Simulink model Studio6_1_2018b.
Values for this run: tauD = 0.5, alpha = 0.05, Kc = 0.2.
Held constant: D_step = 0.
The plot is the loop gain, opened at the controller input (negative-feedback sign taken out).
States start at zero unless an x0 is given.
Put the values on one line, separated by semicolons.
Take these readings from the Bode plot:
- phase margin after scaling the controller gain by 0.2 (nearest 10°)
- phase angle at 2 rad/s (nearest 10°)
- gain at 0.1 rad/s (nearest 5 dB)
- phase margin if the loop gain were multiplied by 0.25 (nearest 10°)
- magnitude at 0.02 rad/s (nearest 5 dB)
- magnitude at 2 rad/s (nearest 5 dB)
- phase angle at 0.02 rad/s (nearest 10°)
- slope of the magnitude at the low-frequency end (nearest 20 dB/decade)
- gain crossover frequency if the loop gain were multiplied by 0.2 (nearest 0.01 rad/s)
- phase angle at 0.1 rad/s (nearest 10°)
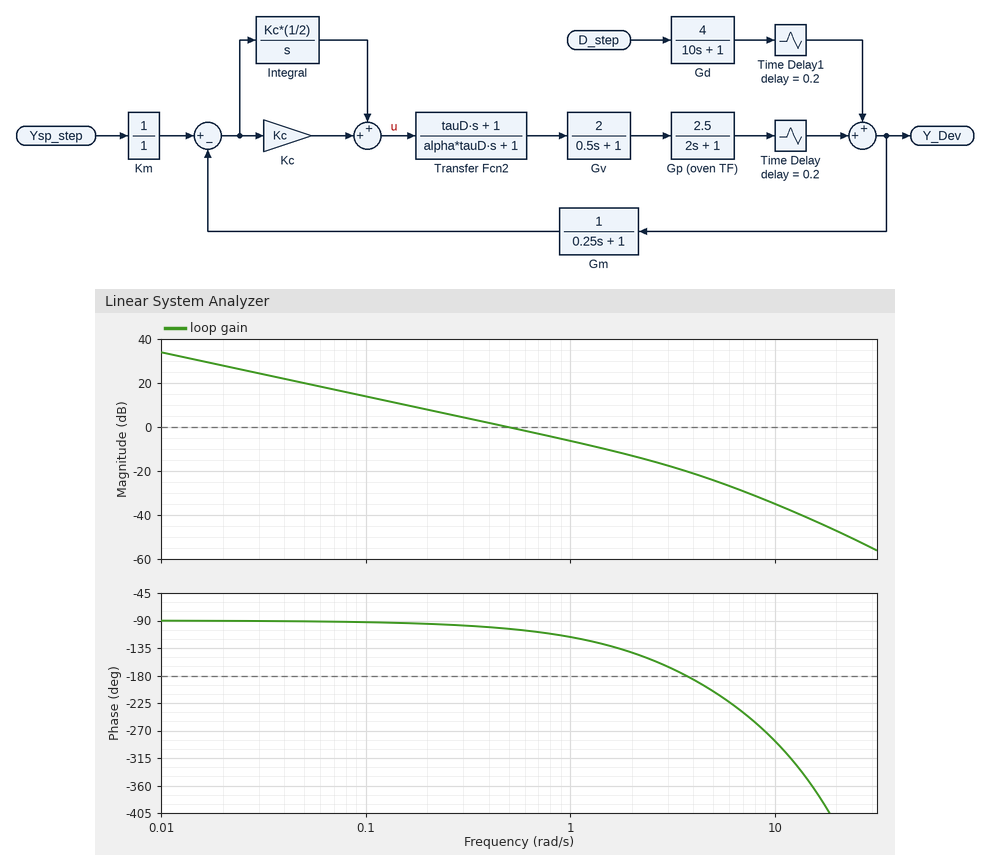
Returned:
90°; -140°; 15 dB; 90°; 30 dB; -15 dB; -90°; -20 dB/decade; 0.10 rad/s; -90°
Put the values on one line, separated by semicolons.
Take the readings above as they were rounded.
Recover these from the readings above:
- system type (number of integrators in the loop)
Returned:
1
